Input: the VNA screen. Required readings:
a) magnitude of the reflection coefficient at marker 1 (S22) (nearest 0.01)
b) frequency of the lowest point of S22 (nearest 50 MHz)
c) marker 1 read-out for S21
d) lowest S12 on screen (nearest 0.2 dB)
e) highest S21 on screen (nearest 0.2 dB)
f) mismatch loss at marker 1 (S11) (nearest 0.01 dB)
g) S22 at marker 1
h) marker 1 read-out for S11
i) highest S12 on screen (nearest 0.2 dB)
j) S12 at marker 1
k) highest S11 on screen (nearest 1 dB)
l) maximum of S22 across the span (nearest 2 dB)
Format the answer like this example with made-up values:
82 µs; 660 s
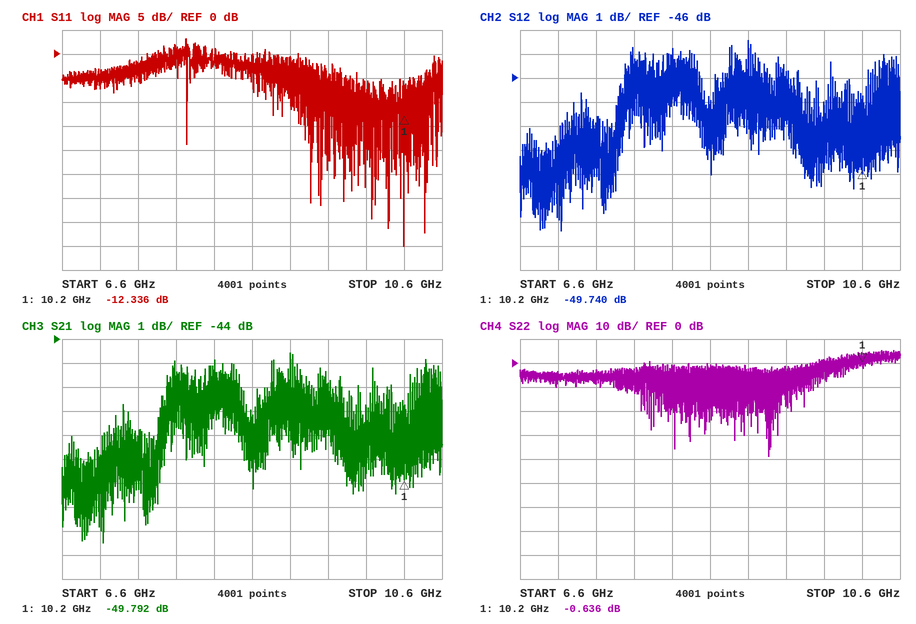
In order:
0.93; 9.20 GHz; -49.792 dB; -52.4 dB; -44.6 dB; 0.26 dB; -0.636 dB; -12.336 dB; -44.4 dB; -49.740 dB; 3 dB; 6 dB
